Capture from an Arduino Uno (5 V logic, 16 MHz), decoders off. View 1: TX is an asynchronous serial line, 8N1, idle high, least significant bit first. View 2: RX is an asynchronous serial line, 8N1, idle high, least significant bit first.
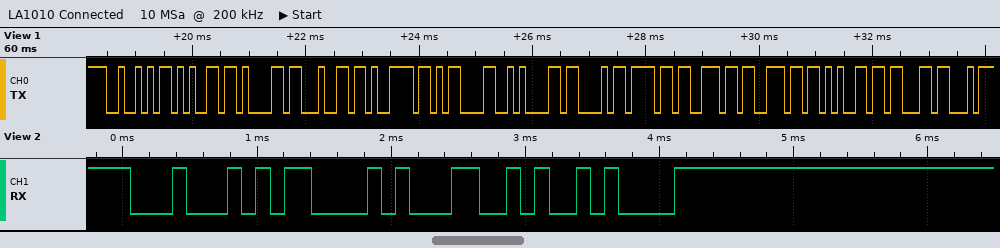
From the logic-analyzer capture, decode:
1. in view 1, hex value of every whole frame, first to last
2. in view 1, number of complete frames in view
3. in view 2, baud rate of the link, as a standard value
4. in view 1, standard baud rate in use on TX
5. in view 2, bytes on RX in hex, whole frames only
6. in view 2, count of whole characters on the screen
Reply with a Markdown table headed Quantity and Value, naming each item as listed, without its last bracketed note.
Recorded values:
| Quantity | Value |
|---|---|
| in view 1, hex value of every whole frame, first to last | 52 65 61 64 79 0D 0A 43 6F 6E 6E 65 63 |
| in view 1, number of complete frames in view | 13 |
| in view 2, baud rate of the link, as a standard value | 9600 baud |
| in view 1, standard baud rate in use on TX | 9600 baud |
| in view 2, bytes on RX in hex, whole frames only | 44 43 4C 0A |
| in view 2, count of whole characters on the screen | 4 |
